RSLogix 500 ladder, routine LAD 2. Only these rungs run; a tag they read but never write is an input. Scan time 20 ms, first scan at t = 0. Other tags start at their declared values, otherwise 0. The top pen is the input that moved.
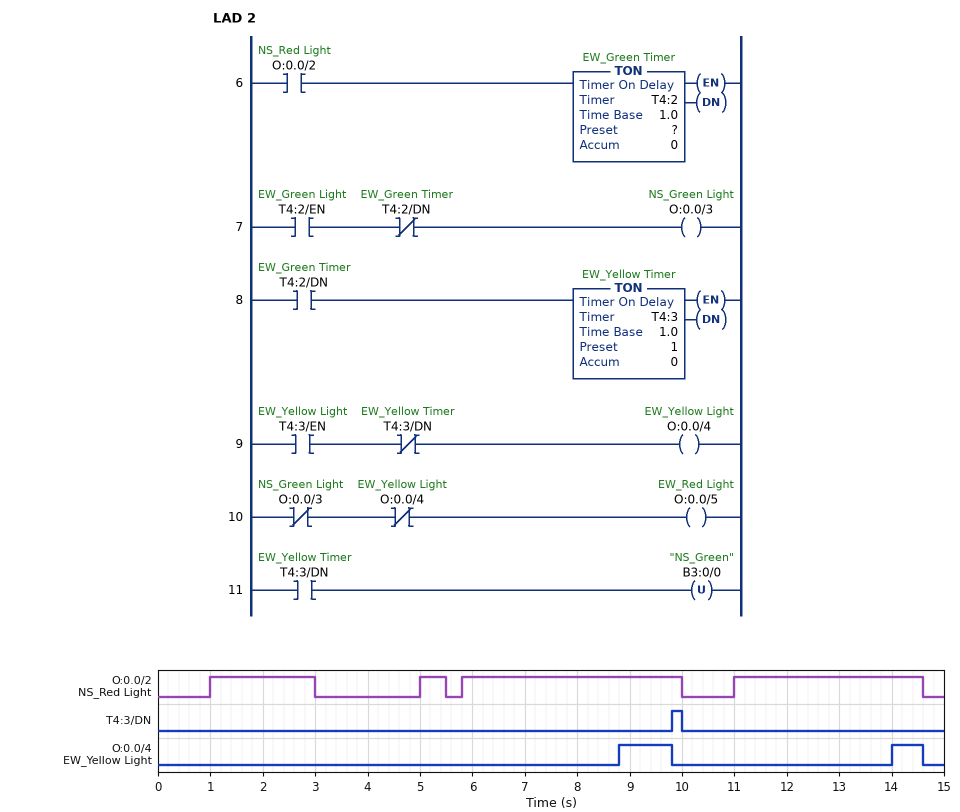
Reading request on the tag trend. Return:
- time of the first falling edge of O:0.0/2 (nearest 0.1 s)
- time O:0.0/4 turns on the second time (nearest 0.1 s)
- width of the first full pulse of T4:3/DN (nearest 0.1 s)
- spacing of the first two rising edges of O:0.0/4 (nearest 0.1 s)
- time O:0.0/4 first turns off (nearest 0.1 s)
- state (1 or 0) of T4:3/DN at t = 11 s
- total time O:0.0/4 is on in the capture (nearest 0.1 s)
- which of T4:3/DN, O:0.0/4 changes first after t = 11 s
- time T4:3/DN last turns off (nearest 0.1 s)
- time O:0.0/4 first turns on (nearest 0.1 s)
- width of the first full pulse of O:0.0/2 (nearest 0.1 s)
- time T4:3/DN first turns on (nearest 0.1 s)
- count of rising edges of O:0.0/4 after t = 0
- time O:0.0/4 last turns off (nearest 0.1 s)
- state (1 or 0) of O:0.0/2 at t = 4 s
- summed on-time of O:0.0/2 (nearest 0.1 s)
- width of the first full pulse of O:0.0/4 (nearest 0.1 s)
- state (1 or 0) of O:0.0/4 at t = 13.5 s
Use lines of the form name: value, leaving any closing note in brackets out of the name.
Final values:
time of the first falling edge of O:0.0/2: 3.0 s
time O:0.0/4 turns on the second time: 14.0 s
width of the first full pulse of T4:3/DN: 0.2 s
spacing of the first two rising edges of O:0.0/4: 5.2 s
time O:0.0/4 first turns off: 9.8 s
state (1 or 0) of T4:3/DN at t = 11 s: 0
total time O:0.0/4 is on in the capture: 1.6 s
which of T4:3/DN, O:0.0/4 changes first after t = 11 s: O:0.0/4
time T4:3/DN last turns off: 10.0 s
time O:0.0/4 first turns on: 8.8 s
width of the first full pulse of O:0.0/2: 2.0 s
time T4:3/DN first turns on: 9.8 s
count of rising edges of O:0.0/4 after t = 0: 2
time O:0.0/4 last turns off: 14.6 s
state (1 or 0) of O:0.0/2 at t = 4 s: 0
summed on-time of O:0.0/2: 10.3 s
width of the first full pulse of O:0.0/4: 1.0 s
state (1 or 0) of O:0.0/4 at t = 13.5 s: 0
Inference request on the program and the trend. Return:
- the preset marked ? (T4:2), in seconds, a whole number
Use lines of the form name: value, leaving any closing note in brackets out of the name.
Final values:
the preset marked ? (T4:2), in seconds, a whole number: 3 s
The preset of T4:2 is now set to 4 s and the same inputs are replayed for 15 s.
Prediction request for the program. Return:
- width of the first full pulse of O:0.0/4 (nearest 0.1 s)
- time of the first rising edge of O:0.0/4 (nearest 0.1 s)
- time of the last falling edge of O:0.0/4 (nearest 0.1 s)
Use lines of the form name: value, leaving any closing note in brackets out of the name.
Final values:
width of the first full pulse of O:0.0/4: 0.2 s
time of the first rising edge of O:0.0/4: 9.8 s
time of the last falling edge of O:0.0/4: 10.0 s
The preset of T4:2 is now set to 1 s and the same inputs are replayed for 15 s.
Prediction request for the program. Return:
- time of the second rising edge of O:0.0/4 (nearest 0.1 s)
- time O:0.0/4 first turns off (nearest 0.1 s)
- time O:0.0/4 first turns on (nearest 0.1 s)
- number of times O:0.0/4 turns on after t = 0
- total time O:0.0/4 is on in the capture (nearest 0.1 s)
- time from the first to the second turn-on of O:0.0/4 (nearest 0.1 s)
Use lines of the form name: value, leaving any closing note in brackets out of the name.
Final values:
time of the second rising edge of O:0.0/4: 6.8 s
time O:0.0/4 first turns off: 3.0 s
time O:0.0/4 first turns on: 2.0 s
number of times O:0.0/4 turns on after t = 0: 3
total time O:0.0/4 is on in the capture: 3.0 s
time from the first to the second turn-on of O:0.0/4: 4.8 s
